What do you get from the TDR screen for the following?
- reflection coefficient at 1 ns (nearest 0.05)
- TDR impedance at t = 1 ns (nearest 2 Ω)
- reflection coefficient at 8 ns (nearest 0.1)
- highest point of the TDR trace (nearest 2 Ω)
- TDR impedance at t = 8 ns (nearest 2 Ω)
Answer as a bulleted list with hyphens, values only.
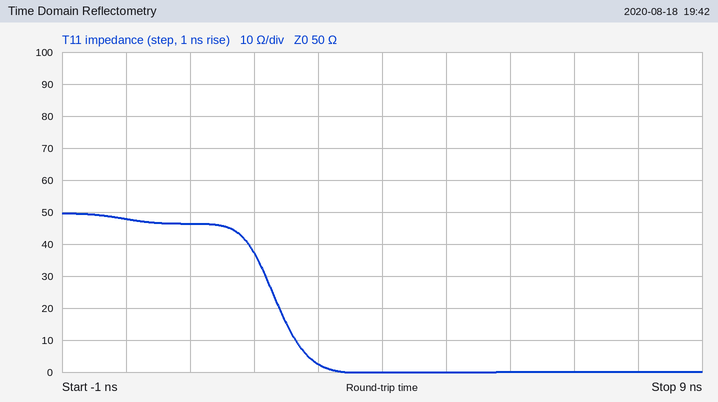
- -0.05
- 46 Ω
- -1.0
- 50 Ω
- 0 Ω
